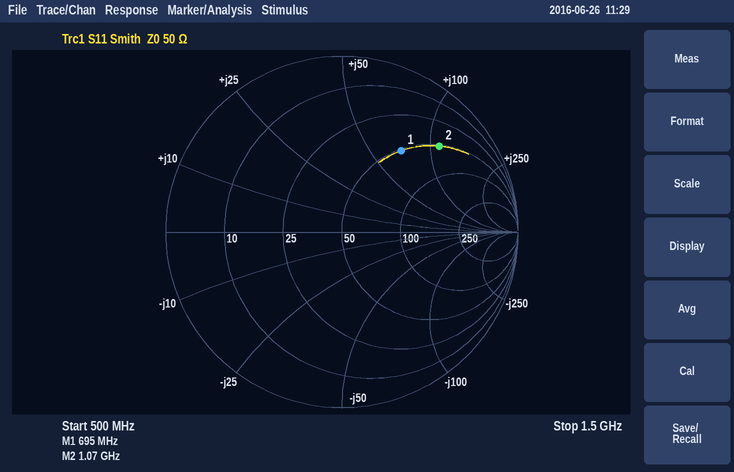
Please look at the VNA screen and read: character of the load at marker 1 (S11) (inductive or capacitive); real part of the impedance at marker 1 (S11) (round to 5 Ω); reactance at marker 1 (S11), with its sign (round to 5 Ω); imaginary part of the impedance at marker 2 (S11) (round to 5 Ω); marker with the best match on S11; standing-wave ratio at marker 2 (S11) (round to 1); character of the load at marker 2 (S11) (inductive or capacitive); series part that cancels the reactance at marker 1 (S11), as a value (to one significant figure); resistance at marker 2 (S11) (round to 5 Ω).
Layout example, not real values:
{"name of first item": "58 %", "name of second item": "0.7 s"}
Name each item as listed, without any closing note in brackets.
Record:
{"character of the load at marker 1 (S11)": "inductive", "real part of the impedance at marker 1 (S11)": "50 Ω", "reactance at marker 1 (S11), with its sign": "+70 Ω", "imaginary part of the impedance at marker 2 (S11)": "+110 Ω", "marker with the best match on S11": "marker 1", "standing-wave ratio at marker 2 (S11)": "7", "character of the load at marker 2 (S11)": "inductive", "series part that cancels the reactance at marker 1 (S11), as a value": "3 pF", "resistance at marker 2 (S11)": "50 Ω"}
